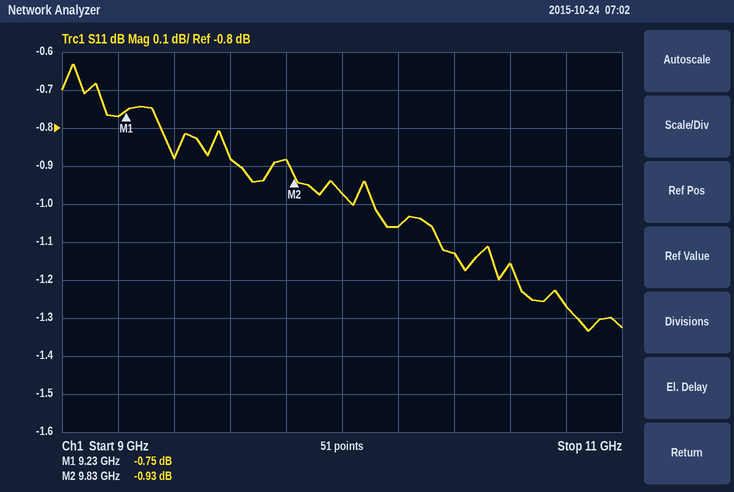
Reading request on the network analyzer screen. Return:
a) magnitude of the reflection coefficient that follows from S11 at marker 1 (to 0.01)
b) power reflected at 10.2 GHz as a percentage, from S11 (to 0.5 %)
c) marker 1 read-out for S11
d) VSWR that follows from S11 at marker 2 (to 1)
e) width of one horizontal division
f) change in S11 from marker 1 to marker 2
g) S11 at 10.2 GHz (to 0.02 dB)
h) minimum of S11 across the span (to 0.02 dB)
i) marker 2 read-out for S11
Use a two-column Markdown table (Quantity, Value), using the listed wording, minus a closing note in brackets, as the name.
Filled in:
| Quantity | Value |
|---|---|
| magnitude of the reflection coefficient that follows from S11 at marker 1 | 0.92 |
| power reflected at 10.2 GHz as a percentage, from S11 | 78.5 % |
| marker 1 read-out for S11 | -0.75 dB |
| VSWR that follows from S11 at marker 2 | 19 |
| width of one horizontal division | 200 MHz |
| change in S11 from marker 1 to marker 2 | -0.18 dB |
| S11 at 10.2 GHz | -1.06 dB |
| minimum of S11 across the span | -1.34 dB |
| marker 2 read-out for S11 | -0.93 dB |
